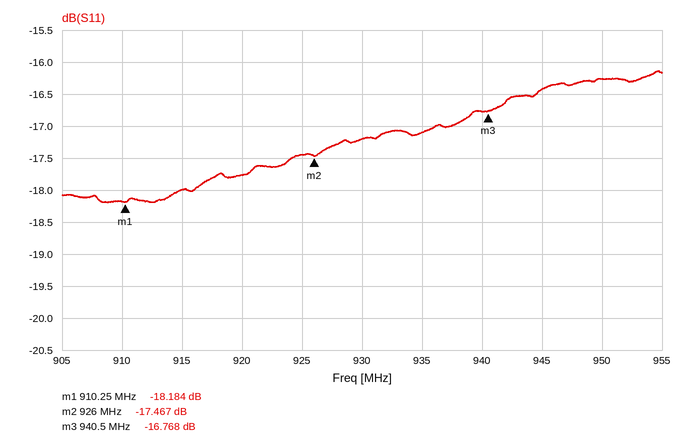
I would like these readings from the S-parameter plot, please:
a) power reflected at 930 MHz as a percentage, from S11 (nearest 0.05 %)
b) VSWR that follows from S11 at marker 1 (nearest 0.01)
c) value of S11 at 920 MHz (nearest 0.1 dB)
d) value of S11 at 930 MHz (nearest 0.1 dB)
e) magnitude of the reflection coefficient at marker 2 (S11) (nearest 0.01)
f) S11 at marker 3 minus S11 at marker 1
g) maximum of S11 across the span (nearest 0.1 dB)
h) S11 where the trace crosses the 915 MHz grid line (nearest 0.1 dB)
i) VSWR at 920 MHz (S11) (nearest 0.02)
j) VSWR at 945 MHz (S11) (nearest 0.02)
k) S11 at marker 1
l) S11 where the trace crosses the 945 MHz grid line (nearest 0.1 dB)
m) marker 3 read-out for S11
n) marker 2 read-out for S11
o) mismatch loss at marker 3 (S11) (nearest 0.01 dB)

1.90 %
1.28
-17.8 dB
-17.2 dB
0.13
1.416 dB
-16.1 dB
-18.0 dB
1.30
1.36
-18.184 dB
-16.4 dB
-16.768 dB
-17.467 dB
0.09 dB
